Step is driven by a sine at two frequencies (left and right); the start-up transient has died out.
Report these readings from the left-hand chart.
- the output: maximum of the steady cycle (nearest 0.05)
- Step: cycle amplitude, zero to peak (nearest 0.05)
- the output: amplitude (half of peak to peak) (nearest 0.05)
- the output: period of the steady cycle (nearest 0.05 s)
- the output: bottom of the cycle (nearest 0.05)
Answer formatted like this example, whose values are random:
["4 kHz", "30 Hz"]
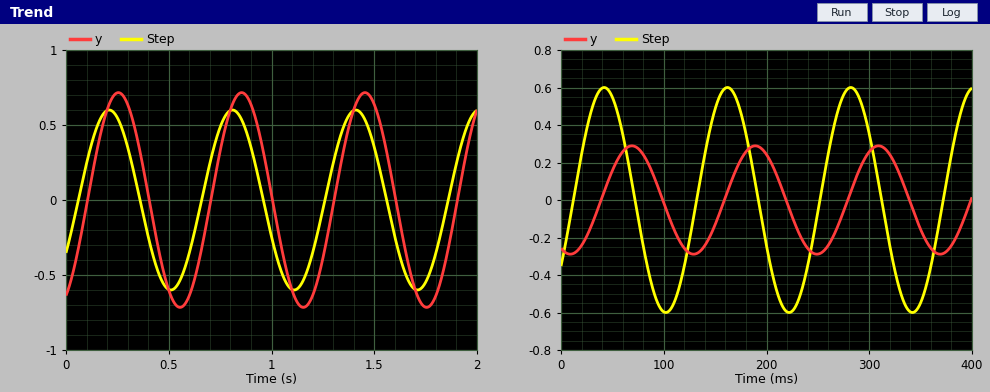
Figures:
["0.70", "0.60", "0.70", "0.60 s", "-0.70"]
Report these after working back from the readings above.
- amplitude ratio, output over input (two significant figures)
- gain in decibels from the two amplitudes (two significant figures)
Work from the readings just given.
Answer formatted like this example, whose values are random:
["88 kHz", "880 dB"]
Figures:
["1.2", "1.3 dB"]
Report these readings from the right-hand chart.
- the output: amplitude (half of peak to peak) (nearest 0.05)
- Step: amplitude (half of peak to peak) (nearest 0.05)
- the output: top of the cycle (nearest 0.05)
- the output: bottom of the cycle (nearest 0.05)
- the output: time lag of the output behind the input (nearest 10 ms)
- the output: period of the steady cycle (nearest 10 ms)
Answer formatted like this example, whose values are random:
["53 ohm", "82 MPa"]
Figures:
["0.30", "0.60", "0.30", "-0.30", "30 ms", "120 ms"]
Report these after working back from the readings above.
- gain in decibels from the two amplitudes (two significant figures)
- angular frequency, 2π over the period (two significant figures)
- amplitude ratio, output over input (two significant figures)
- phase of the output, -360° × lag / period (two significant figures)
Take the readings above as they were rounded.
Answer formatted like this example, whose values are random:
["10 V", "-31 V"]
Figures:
["-6.0 dB", "0.052 rad/ms", "0.50", "-90°"]
